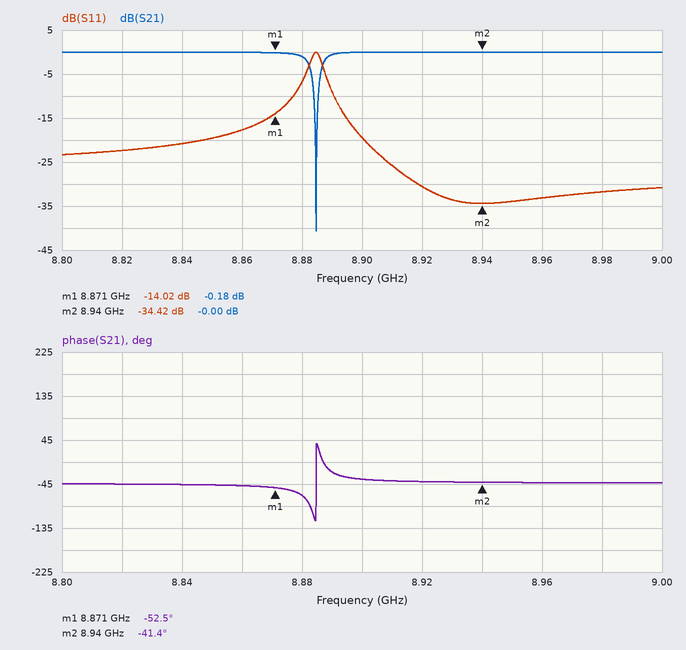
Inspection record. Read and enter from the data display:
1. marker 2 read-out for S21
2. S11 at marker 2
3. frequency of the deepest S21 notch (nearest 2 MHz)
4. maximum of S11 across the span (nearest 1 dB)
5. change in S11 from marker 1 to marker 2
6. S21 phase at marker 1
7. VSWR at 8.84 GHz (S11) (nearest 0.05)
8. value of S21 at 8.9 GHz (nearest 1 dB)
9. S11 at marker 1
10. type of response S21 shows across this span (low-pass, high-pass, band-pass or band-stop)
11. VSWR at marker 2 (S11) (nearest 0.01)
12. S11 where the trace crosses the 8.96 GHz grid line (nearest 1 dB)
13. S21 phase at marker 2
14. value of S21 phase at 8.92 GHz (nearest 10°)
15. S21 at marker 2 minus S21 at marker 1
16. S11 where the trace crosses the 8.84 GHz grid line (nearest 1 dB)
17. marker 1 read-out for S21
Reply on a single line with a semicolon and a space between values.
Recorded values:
-0.00 dB; -34.42 dB; 8.884 GHz; 0 dB; -20.40 dB; -52.5°; 1.20; 0 dB; -14.02 dB; band-stop; 1.04; -33 dB; -41.4°; -40°; 0.18 dB; -21 dB; -0.18 dB
